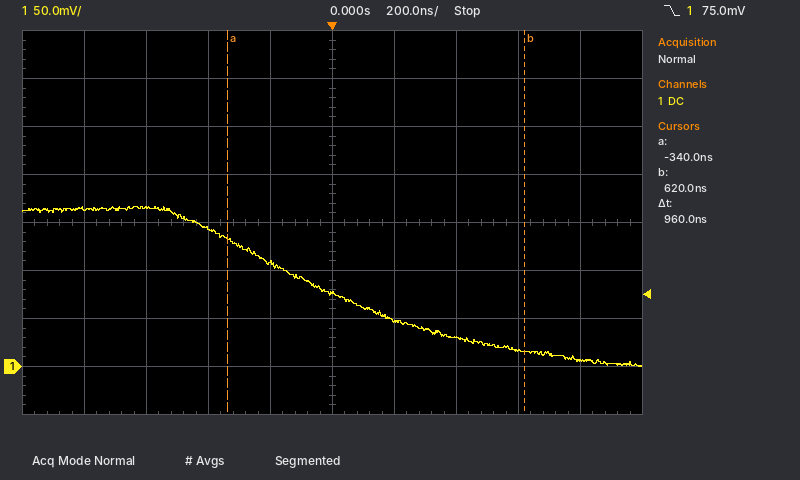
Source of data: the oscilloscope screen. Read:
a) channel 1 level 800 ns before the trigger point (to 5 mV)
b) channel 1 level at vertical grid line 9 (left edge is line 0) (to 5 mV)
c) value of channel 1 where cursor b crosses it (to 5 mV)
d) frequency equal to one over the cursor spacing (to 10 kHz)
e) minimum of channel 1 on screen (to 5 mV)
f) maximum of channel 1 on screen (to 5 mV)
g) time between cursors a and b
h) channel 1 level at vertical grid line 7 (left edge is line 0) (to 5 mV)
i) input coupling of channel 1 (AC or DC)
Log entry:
165 mV
5 mV
15 mV
1.04 MHz
0 mV
165 mV
960 ns
30 mV
DC
